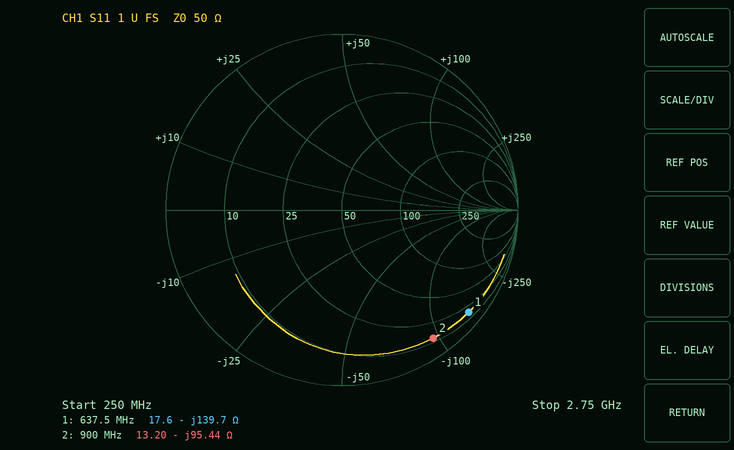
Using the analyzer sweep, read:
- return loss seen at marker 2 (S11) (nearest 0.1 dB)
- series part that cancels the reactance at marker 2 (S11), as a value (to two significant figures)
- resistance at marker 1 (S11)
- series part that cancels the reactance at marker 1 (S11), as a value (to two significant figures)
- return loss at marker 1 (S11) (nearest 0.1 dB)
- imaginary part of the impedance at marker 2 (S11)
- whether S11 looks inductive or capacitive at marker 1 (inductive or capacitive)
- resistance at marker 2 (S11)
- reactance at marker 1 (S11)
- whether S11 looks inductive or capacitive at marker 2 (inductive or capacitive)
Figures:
1.0 dB
17 nH
17.6 Ω
35 nH
0.7 dB
-95.44 Ω
capacitive
13.20 Ω
-139.7 Ω
capacitive
